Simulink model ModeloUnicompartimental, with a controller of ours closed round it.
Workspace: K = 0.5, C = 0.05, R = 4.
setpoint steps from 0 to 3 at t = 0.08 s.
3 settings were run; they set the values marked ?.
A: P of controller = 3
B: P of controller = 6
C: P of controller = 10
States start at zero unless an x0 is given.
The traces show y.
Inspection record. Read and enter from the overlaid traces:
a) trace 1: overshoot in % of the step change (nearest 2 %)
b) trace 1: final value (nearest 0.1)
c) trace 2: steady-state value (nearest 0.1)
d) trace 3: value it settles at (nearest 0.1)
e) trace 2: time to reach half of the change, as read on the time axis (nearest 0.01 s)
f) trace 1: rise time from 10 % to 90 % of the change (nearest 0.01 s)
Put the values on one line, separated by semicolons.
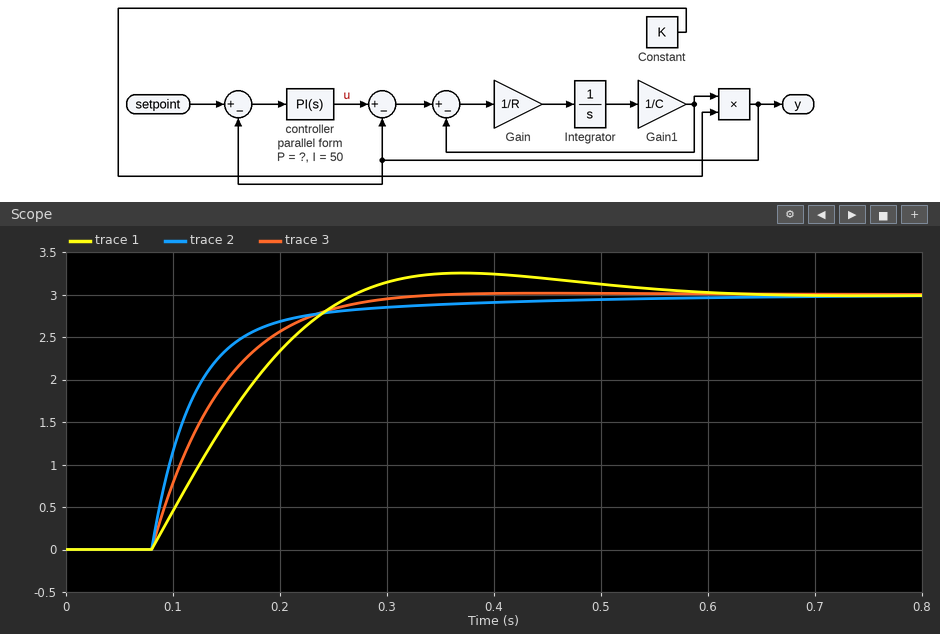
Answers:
8 %; 3.0; 3.0; 3.0; 0.11 s; 0.14 s
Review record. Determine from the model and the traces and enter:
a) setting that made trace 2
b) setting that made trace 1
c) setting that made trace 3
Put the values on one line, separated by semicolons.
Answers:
C; A; B
